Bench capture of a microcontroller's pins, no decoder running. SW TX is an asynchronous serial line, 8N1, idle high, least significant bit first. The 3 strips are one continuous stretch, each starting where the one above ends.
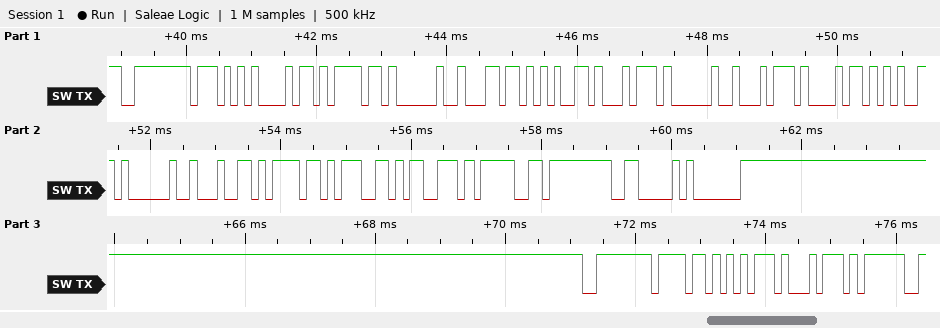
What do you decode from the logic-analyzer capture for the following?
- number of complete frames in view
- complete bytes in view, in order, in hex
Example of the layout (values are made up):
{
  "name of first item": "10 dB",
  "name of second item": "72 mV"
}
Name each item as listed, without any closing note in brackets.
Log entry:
{
  "number of complete frames in view": "26",
  "complete bytes in view, in order, in hex": "FE 57 68 6F 20 6C 65 74 20 74 68 65 20 64 6F 67 73 9F FF 06 01 FE 6F 75 74 3F"
}
